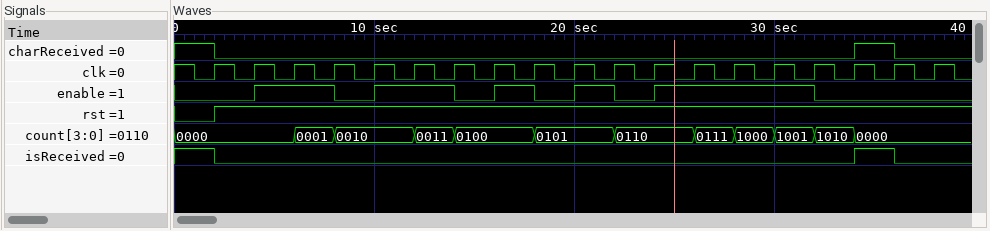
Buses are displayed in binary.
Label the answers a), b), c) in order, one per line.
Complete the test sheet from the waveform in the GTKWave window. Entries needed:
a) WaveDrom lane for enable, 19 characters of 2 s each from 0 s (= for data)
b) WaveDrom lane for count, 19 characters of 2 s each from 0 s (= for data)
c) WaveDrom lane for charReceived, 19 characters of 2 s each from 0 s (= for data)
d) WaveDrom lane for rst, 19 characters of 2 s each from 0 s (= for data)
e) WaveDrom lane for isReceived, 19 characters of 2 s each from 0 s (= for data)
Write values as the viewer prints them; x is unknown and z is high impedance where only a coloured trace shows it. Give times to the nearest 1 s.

a) {name: 'enable', wave: '0.1.01.010101...0..'}
b) {name: 'count', wave: '=..==.==.=.=.=====.', data: '0000 0001 0010 0011 0100 0101 0110 0111 1000 1001 1010 0000'}
c) {name: 'charReceived', wave: '10...............10'}
d) {name: 'rst', wave: '01.................'}
e) {name: 'isReceived', wave: '10...............10'}
